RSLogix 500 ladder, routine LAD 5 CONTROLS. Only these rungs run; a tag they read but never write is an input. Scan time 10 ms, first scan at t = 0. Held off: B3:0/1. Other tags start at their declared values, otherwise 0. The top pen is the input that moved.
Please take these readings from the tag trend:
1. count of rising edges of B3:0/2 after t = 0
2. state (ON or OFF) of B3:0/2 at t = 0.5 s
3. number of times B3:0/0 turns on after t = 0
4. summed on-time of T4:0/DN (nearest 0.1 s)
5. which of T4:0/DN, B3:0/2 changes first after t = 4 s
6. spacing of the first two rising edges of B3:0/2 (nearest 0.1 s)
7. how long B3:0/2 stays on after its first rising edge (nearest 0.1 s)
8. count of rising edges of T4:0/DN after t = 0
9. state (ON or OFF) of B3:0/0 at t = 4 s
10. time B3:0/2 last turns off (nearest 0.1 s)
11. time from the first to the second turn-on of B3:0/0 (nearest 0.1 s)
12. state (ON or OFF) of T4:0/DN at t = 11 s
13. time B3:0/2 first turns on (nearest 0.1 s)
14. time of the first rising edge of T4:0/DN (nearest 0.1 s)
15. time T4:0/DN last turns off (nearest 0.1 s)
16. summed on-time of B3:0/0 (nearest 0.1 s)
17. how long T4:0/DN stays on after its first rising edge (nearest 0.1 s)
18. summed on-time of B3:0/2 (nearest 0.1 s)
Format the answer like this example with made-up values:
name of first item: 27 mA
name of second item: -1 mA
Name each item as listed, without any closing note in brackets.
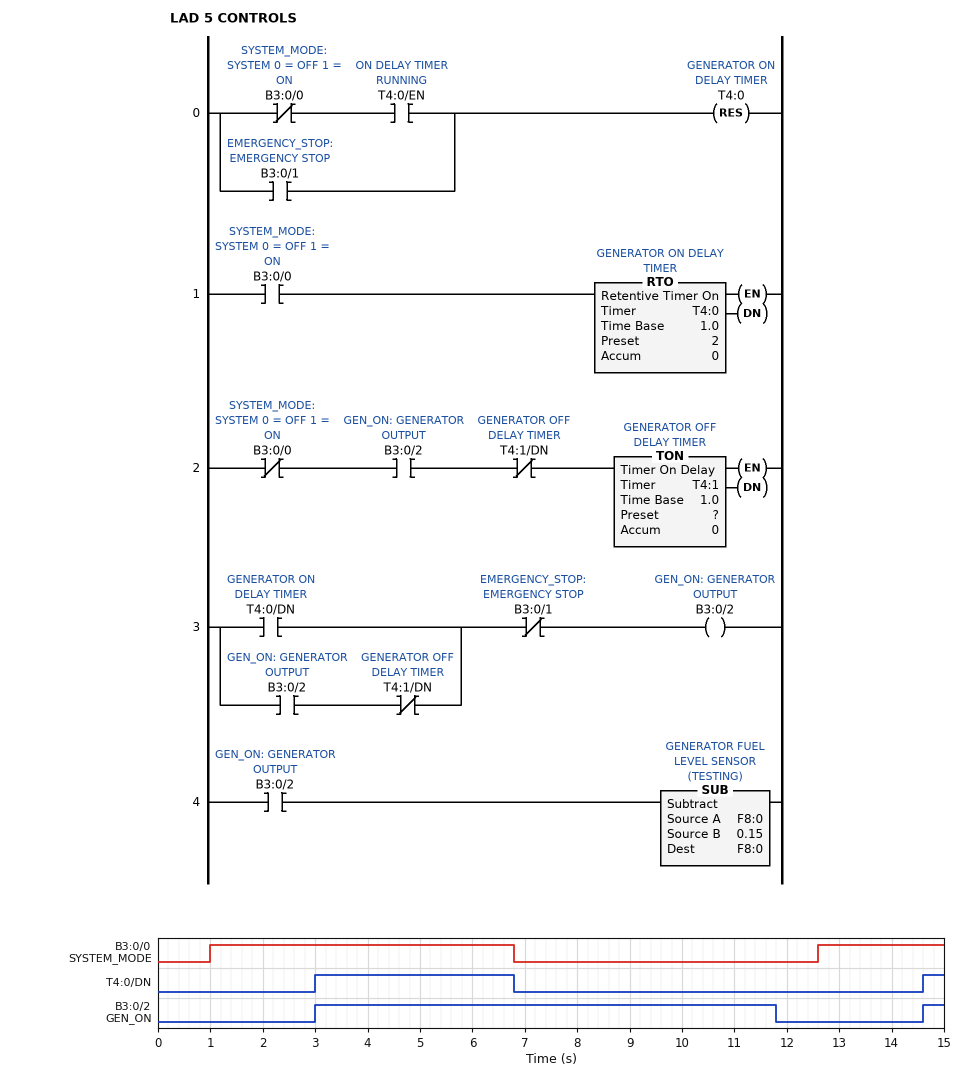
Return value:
count of rising edges of B3:0/2 after t = 0: 2
state (ON or OFF) of B3:0/2 at t = 0.5 s: OFF
number of times B3:0/0 turns on after t = 0: 2
summed on-time of T4:0/DN: 4.2 s
which of T4:0/DN, B3:0/2 changes first after t = 4 s: T4:0/DN
spacing of the first two rising edges of B3:0/2: 11.6 s
how long B3:0/2 stays on after its first rising edge: 8.8 s
count of rising edges of T4:0/DN after t = 0: 2
state (ON or OFF) of B3:0/0 at t = 4 s: ON
time B3:0/2 last turns off: 11.8 s
time from the first to the second turn-on of B3:0/0: 11.6 s
state (ON or OFF) of T4:0/DN at t = 11 s: OFF
time B3:0/2 first turns on: 3.0 s
time of the first rising edge of T4:0/DN: 3.0 s
time T4:0/DN last turns off: 6.8 s
summed on-time of B3:0/0: 8.2 s
how long T4:0/DN stays on after its first rising edge: 3.8 s
summed on-time of B3:0/2: 9.2 s
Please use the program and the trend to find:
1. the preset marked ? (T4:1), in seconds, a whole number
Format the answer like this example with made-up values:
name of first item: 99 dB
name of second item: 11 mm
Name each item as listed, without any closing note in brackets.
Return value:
the preset marked ? (T4:1), in seconds, a whole number: 5 s
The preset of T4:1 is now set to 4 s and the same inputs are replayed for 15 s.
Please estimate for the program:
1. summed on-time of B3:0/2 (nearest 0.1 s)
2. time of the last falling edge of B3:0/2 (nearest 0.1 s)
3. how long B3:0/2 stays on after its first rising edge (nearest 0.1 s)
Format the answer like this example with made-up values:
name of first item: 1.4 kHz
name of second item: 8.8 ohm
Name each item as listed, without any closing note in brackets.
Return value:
summed on-time of B3:0/2: 8.2 s
time of the last falling edge of B3:0/2: 10.8 s
how long B3:0/2 stays on after its first rising edge: 7.8 s
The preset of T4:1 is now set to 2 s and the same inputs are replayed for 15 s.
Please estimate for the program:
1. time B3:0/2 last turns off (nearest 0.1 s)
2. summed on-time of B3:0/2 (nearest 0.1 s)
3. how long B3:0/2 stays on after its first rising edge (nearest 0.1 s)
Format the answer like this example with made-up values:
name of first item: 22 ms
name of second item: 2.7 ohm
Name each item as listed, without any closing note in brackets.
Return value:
time B3:0/2 last turns off: 8.8 s
summed on-time of B3:0/2: 6.2 s
how long B3:0/2 stays on after its first rising edge: 5.8 s
